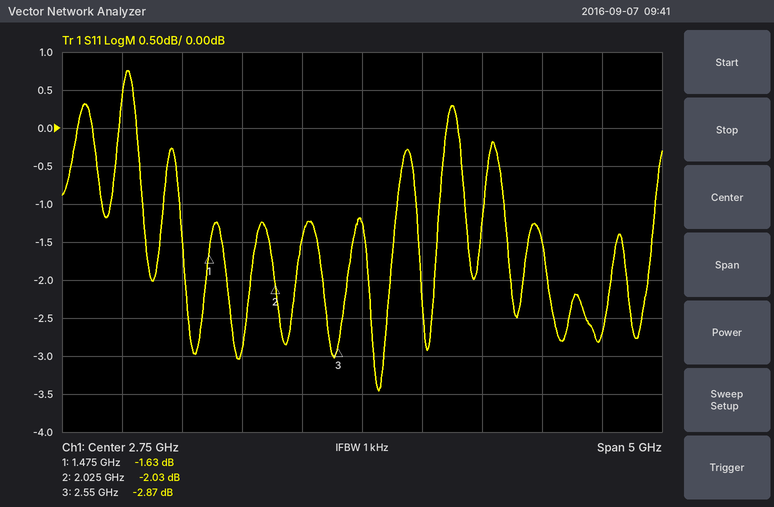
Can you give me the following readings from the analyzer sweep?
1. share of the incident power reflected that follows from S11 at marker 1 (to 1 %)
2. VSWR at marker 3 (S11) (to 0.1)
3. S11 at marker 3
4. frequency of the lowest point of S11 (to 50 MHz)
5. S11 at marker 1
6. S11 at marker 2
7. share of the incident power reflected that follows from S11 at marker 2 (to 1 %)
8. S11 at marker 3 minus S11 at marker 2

69 %
6.1
-2.87 dB
2.90 GHz
-1.63 dB
-2.03 dB
63 %
-0.84 dB
